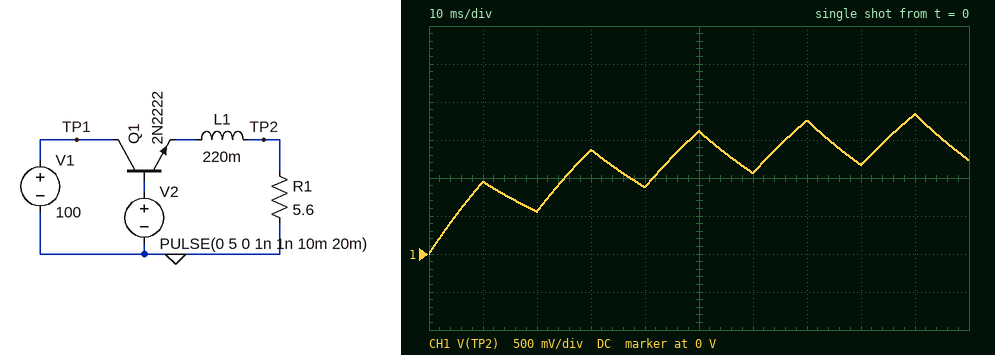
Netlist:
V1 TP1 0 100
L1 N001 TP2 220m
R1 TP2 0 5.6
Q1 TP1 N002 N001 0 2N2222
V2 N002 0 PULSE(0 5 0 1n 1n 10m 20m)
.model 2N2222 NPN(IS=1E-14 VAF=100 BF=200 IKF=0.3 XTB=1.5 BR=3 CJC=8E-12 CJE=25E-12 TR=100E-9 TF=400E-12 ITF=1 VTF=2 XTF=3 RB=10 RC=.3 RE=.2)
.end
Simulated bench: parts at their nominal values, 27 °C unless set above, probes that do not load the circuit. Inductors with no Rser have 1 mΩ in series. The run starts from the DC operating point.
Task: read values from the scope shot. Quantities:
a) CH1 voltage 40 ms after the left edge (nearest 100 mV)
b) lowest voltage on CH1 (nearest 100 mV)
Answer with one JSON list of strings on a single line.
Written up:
["900 mV", "0 V"]
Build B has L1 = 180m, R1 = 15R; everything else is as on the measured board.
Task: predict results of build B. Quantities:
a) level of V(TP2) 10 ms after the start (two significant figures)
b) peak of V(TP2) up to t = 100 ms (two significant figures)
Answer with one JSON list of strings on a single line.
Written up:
["2.4 V", "2.7 V"]
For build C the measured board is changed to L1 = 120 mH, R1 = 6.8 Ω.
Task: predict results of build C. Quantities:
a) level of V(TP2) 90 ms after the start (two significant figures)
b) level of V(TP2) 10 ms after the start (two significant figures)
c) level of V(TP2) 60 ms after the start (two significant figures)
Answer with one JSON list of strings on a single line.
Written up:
["2.3 V", "1.8 V", "940 mV"]
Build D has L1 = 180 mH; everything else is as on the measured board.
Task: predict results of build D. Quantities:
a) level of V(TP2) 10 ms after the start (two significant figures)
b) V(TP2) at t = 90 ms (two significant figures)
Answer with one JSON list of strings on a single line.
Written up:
["1.1 V", "2.0 V"]
